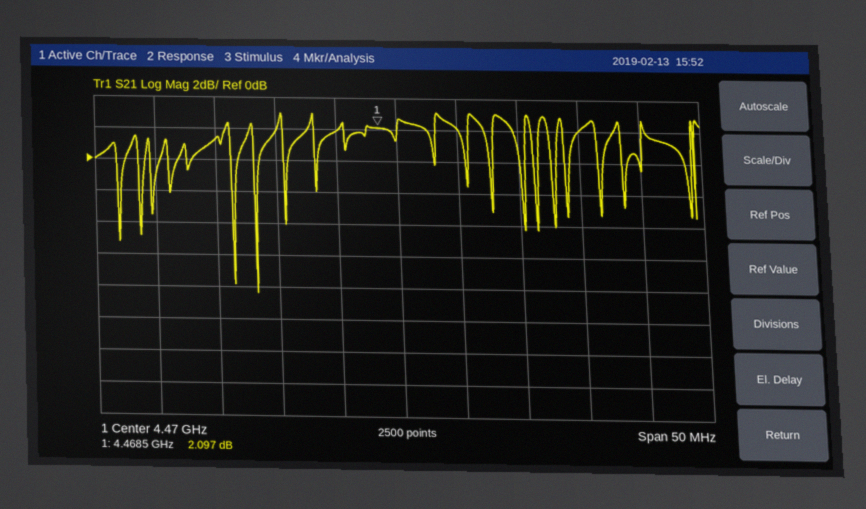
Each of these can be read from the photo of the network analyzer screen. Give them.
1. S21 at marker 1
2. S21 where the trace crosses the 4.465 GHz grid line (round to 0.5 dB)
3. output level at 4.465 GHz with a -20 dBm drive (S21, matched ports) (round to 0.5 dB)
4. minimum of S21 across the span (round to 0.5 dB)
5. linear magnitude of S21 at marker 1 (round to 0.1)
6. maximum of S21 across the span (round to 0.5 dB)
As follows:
2.097 dB
2.0 dB
-18.0 dBm
-8.5 dB
1.3
3.0 dB
